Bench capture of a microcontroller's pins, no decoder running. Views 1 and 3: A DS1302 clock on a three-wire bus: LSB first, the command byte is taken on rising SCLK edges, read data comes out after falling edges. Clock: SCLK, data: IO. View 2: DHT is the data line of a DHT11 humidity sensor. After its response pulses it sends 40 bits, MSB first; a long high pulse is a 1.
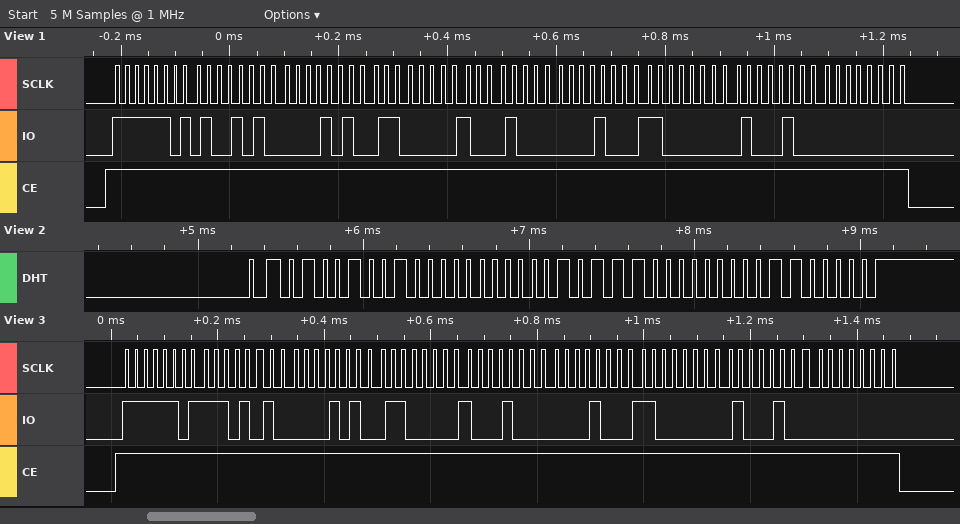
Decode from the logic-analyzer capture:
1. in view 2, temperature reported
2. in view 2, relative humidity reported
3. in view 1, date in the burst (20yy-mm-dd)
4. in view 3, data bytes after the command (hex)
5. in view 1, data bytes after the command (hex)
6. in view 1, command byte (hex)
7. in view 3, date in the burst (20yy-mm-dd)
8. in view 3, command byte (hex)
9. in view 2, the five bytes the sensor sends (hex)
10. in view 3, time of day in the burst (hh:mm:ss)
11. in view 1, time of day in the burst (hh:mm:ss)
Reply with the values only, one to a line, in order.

23.0 °C
73 %
2022-10-11
57 50 06 11 10 03 22 00
52 50 06 11 10 03 22 00
0xBF
2022-10-11
0xBF
49 00 17 00 60
06:50:57
06:50:52
